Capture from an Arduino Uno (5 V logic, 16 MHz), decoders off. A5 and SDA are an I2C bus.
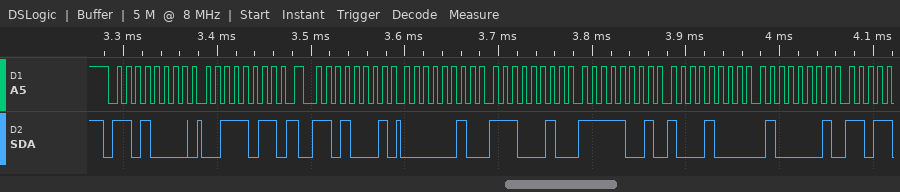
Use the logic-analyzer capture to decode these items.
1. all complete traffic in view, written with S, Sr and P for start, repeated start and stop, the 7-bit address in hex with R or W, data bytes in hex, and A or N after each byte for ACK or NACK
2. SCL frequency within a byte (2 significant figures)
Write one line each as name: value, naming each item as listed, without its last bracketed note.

all complete traffic in view, written with S, Sr and P for start, repeated start and stop, the 7-bit address in hex with R or W, data bytes in hex, and A or N after each byte for ACK or NACK: S 68W A 3B A Sr 68R A 02 A E2 A F9 A 88 A 41 A
SCL frequency within a byte: 100 kHz
